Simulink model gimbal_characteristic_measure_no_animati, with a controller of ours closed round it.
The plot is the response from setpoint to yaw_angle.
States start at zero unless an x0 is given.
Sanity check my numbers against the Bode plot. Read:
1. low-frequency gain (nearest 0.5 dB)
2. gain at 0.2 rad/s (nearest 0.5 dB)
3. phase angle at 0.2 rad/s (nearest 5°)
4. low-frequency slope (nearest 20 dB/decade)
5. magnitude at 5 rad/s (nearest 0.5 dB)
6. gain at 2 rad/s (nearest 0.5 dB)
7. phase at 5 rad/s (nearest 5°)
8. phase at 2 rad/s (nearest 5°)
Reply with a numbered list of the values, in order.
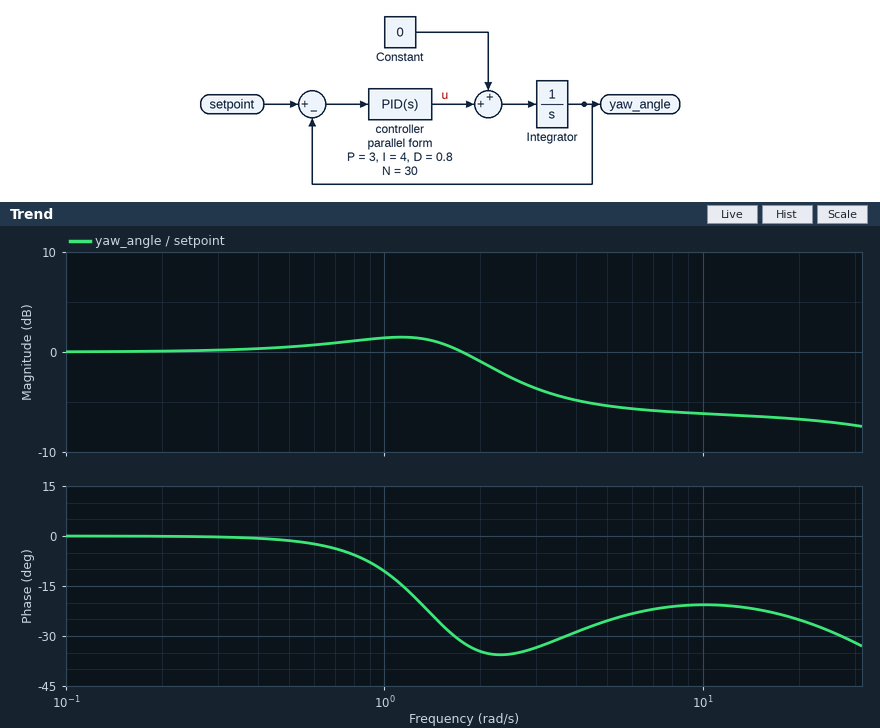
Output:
1. 0.0 dB
2. 0.0 dB
3. 0°
4. 0 dB/decade
5. -5.5 dB
6. -1.0 dB
7. -25°
8. -35°
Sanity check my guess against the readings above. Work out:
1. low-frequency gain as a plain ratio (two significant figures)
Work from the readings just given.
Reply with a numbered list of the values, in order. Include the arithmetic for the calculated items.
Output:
1. 10^(0 / 20) = 1.0
